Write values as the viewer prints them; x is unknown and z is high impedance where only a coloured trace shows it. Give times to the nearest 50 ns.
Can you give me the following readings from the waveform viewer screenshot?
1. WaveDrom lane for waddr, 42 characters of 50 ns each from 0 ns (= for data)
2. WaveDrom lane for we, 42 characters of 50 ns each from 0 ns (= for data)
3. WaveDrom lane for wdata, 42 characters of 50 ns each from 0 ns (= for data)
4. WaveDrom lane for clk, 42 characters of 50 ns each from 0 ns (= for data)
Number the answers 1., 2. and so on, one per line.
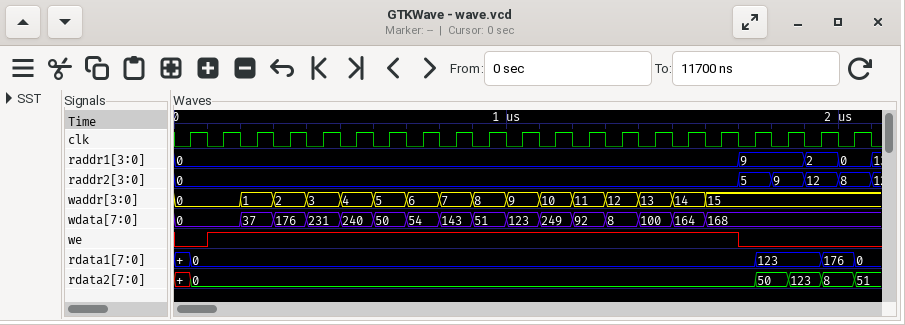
1. {name: 'waddr', wave: '=...=.=.=.=.=.=.=.=.=.=.=.=.=.=.=.........', data: '0 1 2 3 4 5 6 7 8 9 10 11 12 13 14 15'}
2. {name: 'we', wave: '0.1...............................0.......'}
3. {name: 'wdata', wave: '=...=.=.=.=.=.=.=.=.=.=.=.=.=.=.=.........', data: '0 37 176 231 240 50 54 143 51 123 249 92 8 100 164 168'}
4. {name: 'clk', wave: '010101010101010101010101010101010101010101'}
